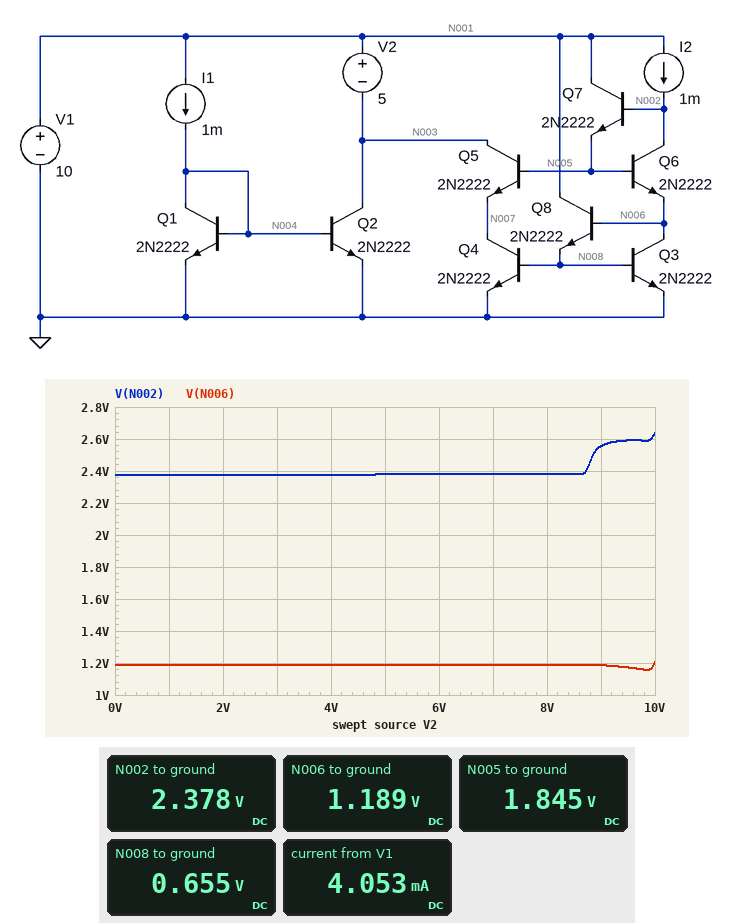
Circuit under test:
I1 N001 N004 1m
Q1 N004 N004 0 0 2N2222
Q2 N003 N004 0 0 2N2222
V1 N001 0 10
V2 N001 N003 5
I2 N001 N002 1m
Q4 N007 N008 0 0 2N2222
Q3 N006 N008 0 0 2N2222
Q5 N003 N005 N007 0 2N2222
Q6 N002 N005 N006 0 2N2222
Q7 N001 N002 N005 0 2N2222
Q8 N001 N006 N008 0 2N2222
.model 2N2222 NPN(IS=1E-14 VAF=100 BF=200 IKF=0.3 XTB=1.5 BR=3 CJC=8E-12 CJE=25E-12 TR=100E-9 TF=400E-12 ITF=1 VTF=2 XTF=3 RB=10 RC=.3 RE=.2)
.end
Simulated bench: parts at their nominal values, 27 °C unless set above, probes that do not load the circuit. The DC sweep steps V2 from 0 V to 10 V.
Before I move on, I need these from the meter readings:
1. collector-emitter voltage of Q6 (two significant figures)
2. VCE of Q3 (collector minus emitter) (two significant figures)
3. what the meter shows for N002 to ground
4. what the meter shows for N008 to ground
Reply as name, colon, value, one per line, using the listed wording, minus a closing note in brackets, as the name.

collector-emitter voltage of Q6: 1.2 V
VCE of Q3 (collector minus emitter): 1.2 V
what the meter shows for N002 to ground: 2.378 V
what the meter shows for N008 to ground: 0.655 V
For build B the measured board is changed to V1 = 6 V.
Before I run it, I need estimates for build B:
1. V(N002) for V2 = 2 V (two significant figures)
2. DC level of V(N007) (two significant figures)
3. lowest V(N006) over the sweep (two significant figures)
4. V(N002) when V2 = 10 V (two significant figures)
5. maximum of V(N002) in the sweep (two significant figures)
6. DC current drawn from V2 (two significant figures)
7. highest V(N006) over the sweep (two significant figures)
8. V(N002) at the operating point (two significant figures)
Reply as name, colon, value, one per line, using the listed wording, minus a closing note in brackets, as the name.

V(N002) for V2 = 2 V: 2.4 V
DC level of V(N007): 1.0 V
lowest V(N006) over the sweep: -2.3 V
V(N002) when V2 = 10 V: -900 mV
maximum of V(N002) in the sweep: 2.7 V
DC current drawn from V2: 7.8 mA
highest V(N006) over the sweep: 1.3 V
V(N002) at the operating point: 2.6 V
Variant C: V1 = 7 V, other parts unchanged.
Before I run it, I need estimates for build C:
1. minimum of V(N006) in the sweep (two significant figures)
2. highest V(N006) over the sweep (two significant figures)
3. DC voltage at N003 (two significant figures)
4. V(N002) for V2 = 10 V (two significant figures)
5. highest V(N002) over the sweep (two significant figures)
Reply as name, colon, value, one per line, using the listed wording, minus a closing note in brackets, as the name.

minimum of V(N006) in the sweep: -1.3 V
highest V(N006) over the sweep: 1.3 V
DC voltage at N003: 2.0 V
V(N002) for V2 = 10 V: 100 mV
highest V(N002) over the sweep: 2.7 V
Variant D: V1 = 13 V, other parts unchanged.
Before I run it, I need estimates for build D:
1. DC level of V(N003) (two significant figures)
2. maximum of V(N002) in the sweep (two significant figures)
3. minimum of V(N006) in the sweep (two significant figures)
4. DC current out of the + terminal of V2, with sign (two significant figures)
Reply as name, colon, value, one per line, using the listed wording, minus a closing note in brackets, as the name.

DC level of V(N003): 8.0 V
maximum of V(N002) in the sweep: 2.4 V
minimum of V(N006) in the sweep: 1.2 V
DC current out of the + terminal of V2, with sign: -2.1 mA
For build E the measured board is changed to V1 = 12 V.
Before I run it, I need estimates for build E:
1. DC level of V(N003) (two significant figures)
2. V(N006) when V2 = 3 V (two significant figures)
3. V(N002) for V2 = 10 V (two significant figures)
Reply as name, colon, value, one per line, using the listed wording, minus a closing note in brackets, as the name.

DC level of V(N003): 7.0 V
V(N006) when V2 = 3 V: 1.2 V
V(N002) for V2 = 10 V: 2.4 V
